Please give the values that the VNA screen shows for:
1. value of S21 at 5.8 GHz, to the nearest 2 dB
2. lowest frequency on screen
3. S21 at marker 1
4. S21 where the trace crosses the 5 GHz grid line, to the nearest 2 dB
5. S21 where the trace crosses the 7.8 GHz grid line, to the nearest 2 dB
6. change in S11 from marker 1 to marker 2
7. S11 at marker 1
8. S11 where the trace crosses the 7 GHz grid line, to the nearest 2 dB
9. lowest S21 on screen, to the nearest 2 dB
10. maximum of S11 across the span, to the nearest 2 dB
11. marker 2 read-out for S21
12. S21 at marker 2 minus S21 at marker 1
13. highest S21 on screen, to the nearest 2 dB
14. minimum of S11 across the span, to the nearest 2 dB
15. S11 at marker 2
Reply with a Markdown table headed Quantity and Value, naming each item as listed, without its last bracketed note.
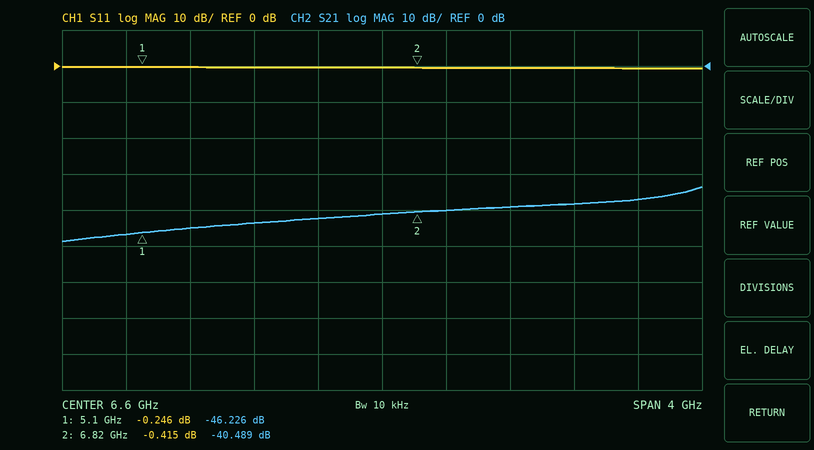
| Quantity | Value |
|---|---|
| value of S21 at 5.8 GHz, to the nearest 2 dB | -44 dB |
| lowest frequency on screen | 4.6 GHz |
| S21 at marker 1 | -46.226 dB |
| S21 where the trace crosses the 5 GHz grid line, to the nearest 2 dB | -46 dB |
| S21 where the trace crosses the 7.8 GHz grid line, to the nearest 2 dB | -38 dB |
| change in S11 from marker 1 to marker 2 | -0.169 dB |
| S11 at marker 1 | -0.246 dB |
| S11 where the trace crosses the 7 GHz grid line, to the nearest 2 dB | 0 dB |
| lowest S21 on screen, to the nearest 2 dB | -48 dB |
| maximum of S11 across the span, to the nearest 2 dB | 0 dB |
| marker 2 read-out for S21 | -40.489 dB |
| S21 at marker 2 minus S21 at marker 1 | 5.737 dB |
| highest S21 on screen, to the nearest 2 dB | -34 dB |
| minimum of S11 across the span, to the nearest 2 dB | 0 dB |
| S11 at marker 2 | -0.415 dB |
